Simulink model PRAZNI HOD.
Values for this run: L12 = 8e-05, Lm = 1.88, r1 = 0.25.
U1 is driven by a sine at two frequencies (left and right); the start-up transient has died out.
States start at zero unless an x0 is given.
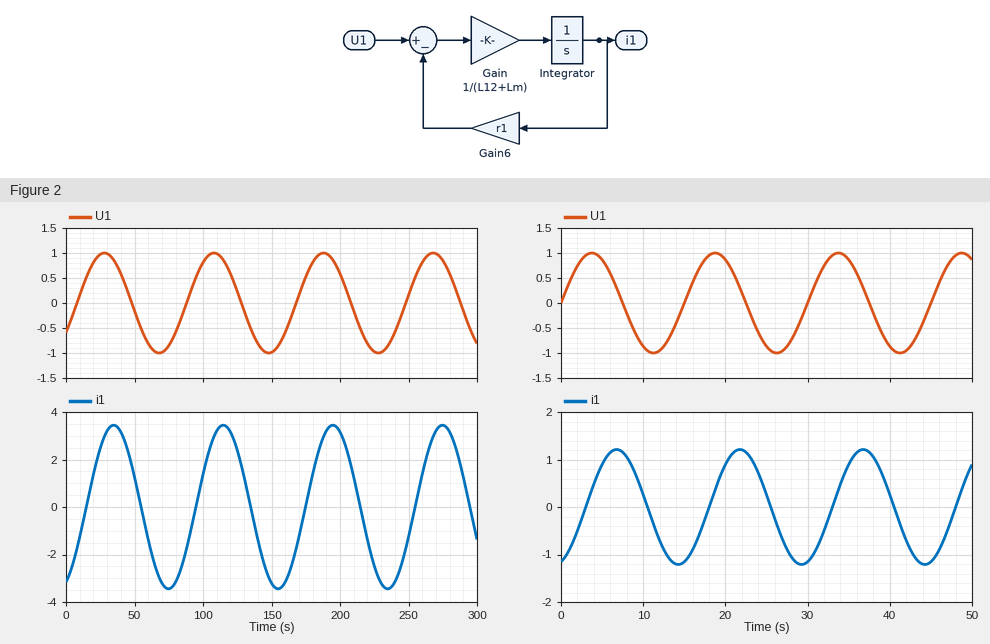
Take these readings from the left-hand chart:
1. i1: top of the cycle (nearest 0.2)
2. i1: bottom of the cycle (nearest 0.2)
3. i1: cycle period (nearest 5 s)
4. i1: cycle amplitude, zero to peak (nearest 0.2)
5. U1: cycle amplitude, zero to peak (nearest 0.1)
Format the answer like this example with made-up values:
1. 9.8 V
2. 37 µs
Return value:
1. 3.4
2. -3.4
3. 80 s
4. 3.4
5. 1.0
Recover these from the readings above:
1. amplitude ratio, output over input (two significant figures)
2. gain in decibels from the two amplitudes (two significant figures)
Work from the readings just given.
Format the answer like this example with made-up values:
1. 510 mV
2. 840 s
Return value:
1. 3.4
2. 11 dB
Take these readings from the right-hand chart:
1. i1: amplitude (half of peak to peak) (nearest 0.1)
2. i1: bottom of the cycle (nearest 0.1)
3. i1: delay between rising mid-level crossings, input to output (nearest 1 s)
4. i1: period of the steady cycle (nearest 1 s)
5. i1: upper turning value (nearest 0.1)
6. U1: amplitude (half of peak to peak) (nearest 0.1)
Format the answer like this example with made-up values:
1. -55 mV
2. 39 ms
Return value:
1. 1.2
2. -1.2
3. 3 s
4. 15 s
5. 1.2
6. 1.0
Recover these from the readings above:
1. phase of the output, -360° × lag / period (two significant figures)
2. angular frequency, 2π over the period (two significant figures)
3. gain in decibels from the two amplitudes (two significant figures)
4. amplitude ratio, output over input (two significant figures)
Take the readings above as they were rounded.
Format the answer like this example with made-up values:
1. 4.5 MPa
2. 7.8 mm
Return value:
1. -72°
2. 0.42 rad/s
3. 1.6 dB
4. 1.2
